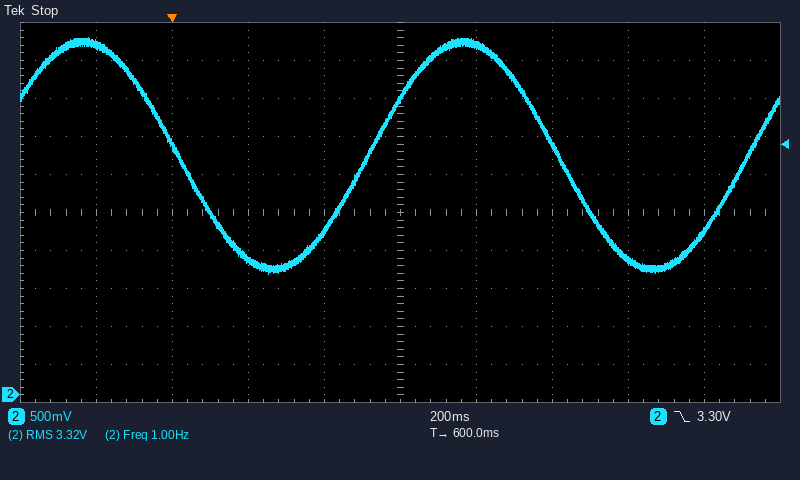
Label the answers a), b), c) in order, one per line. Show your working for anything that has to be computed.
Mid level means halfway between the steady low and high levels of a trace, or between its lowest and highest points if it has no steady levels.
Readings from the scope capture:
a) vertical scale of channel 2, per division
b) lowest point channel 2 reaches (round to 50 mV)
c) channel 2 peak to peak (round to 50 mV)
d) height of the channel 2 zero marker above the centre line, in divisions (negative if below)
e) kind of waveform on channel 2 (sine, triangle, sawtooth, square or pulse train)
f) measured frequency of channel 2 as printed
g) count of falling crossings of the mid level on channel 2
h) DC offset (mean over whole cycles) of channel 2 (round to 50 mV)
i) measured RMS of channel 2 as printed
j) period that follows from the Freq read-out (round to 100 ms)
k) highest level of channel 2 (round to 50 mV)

a) 500 mV
b) 1.60 V
c) 4.70 V − (1.60 V) = 3.10 V
d) -4.8 div
e) sine
f) 1.00 Hz
g) 2
h) (4.70 V + (1.60 V)) / 2 ≈ 3.15 V
i) 3.32 V
j) 1 / 1.00 Hz ≈ 1.0 s
k) 4.70 V
